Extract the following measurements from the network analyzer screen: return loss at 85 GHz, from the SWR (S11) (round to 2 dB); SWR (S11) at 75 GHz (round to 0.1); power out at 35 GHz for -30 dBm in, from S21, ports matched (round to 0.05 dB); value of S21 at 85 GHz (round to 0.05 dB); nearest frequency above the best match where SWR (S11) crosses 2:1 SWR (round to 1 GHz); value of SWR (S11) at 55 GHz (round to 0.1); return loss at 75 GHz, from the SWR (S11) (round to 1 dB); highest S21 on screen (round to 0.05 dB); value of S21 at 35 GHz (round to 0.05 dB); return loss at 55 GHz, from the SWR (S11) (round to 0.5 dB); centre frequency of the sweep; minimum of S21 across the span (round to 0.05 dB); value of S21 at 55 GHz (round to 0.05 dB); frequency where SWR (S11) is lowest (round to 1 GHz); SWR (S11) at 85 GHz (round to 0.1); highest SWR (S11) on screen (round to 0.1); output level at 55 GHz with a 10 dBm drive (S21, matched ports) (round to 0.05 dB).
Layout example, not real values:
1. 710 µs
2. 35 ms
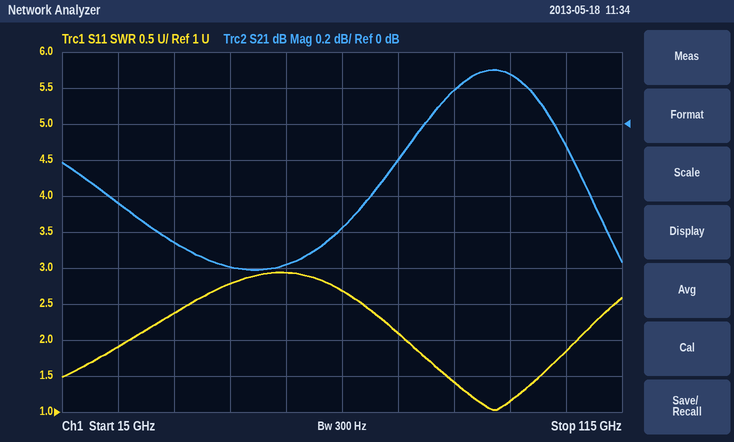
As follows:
1. 16 dB
2. 2.1
3. -30.65 dBm
4. 0.20 dB
5. 107 GHz
6. 2.9
7. 9 dB
8. 0.30 dB
9. -0.65 dB
10. 6.0 dB
11. 65 GHz
12. -0.80 dB
13. -0.80 dB
14. 92 GHz
15. 1.4
16. 2.9
17. 9.20 dBm
